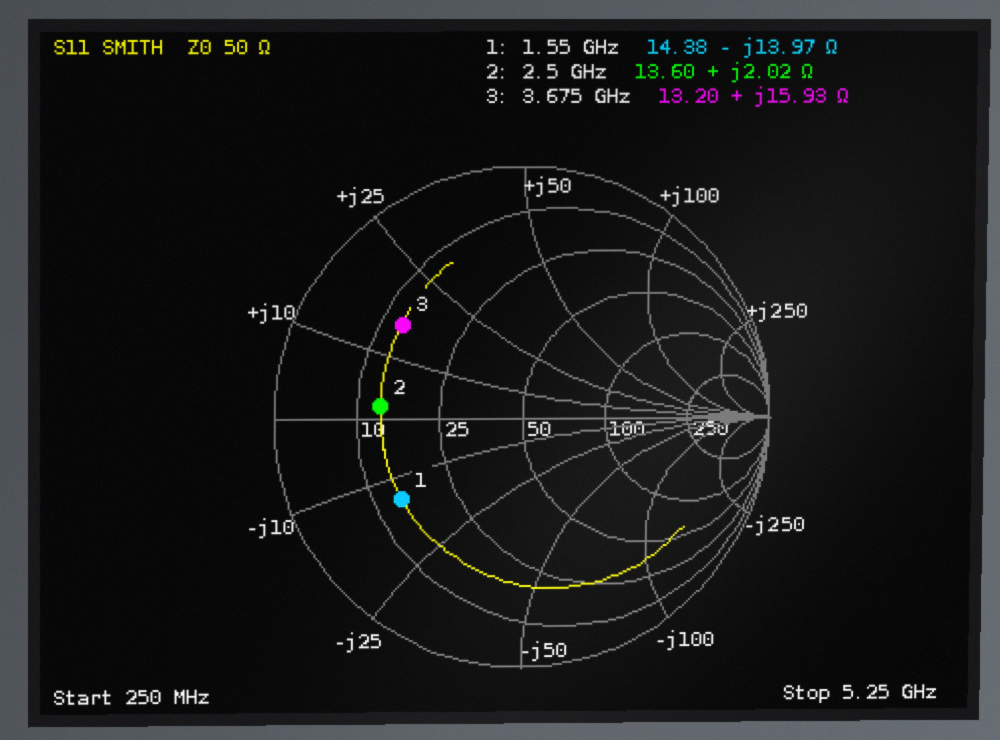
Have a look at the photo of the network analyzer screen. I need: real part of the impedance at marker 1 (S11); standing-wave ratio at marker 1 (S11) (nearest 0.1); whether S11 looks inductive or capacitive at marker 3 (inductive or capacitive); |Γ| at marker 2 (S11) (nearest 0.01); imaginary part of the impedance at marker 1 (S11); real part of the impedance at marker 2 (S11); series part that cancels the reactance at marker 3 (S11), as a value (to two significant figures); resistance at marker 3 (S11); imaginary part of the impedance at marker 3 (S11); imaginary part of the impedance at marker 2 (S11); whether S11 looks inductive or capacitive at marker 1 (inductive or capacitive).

14.38 Ω
3.8
inductive
0.57
-13.97 Ω
13.60 Ω
2.7 pF
13.20 Ω
+15.93 Ω
+2.02 Ω
capacitive
